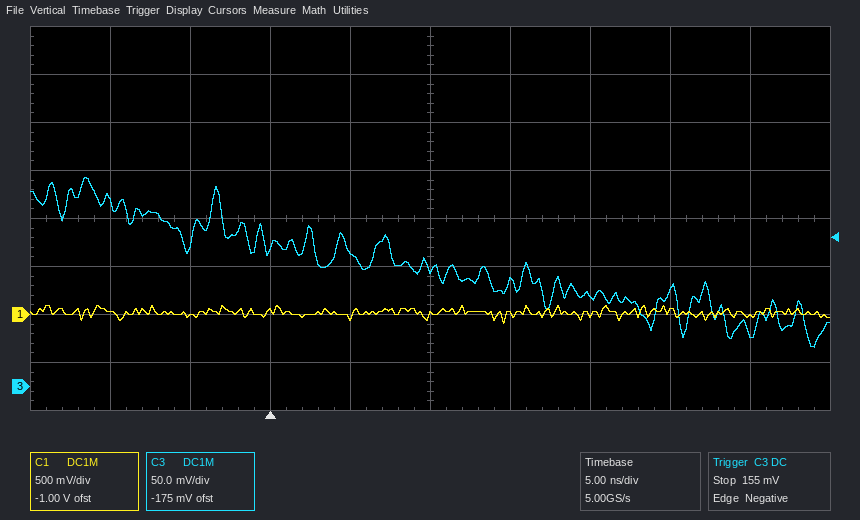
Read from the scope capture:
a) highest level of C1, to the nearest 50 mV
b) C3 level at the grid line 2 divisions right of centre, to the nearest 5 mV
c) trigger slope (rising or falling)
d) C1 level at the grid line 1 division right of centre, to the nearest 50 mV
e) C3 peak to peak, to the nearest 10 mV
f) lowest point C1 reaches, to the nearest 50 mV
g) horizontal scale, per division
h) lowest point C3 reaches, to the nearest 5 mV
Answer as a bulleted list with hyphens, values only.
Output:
- 100 mV
- 95 mV
- falling
- 0 mV
- 180 mV
- -100 mV
- 5 ns
- 40 mV
